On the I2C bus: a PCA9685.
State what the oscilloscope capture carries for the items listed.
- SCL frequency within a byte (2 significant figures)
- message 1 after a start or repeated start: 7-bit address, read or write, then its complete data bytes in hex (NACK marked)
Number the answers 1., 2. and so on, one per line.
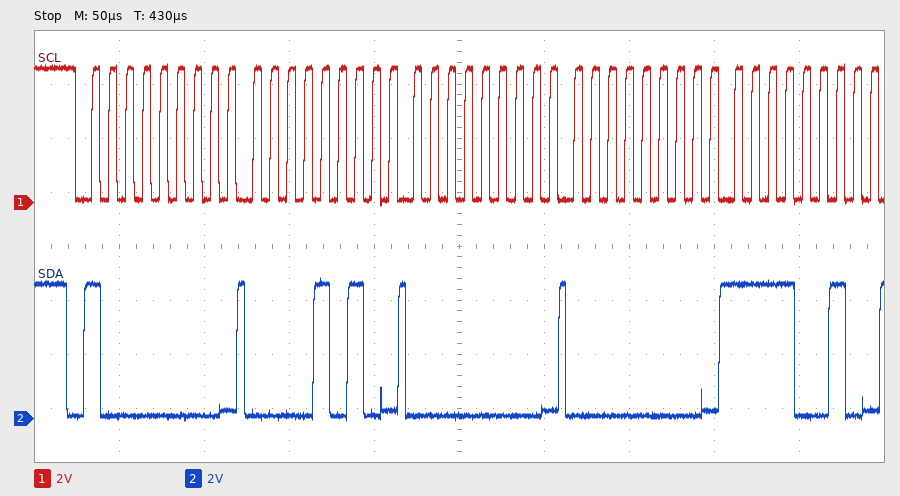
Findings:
1. 100 kHz
2. 0x40 write: 0A 00 00 F2
